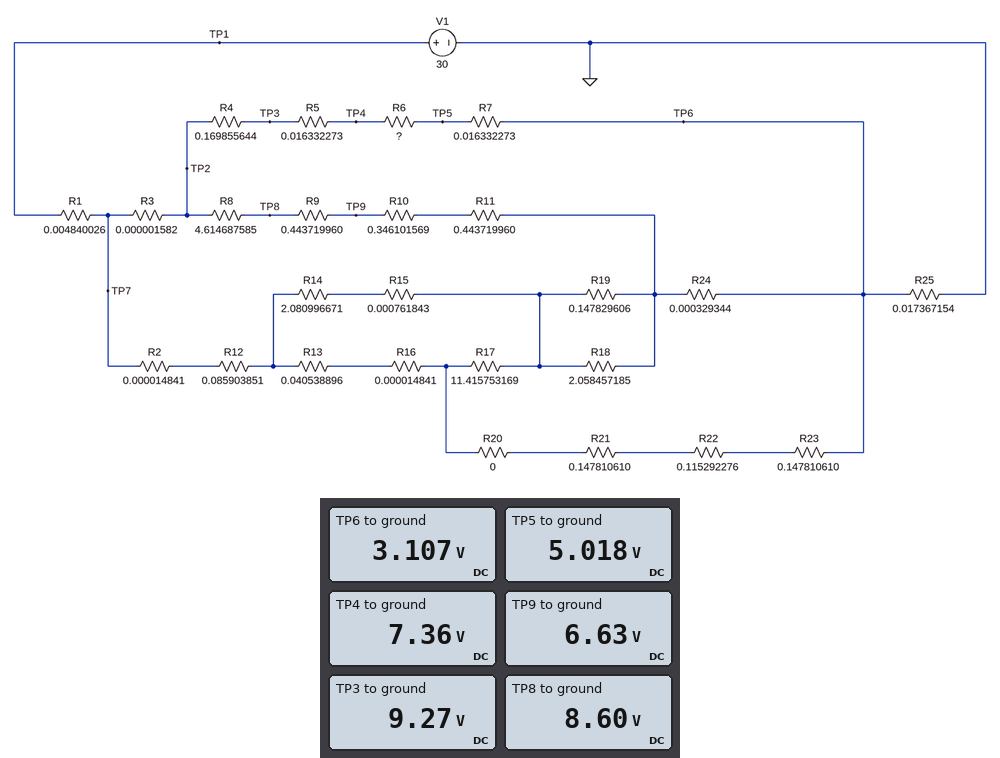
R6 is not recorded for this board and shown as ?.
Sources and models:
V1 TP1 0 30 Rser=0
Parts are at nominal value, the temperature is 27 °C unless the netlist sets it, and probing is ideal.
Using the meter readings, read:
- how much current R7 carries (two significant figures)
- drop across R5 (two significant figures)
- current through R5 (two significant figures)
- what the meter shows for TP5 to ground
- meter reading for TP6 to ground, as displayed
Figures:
120 A
1.9 V
120 A
5.018 V
3.107 V
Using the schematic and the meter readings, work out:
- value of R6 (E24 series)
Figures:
0.02 Ω
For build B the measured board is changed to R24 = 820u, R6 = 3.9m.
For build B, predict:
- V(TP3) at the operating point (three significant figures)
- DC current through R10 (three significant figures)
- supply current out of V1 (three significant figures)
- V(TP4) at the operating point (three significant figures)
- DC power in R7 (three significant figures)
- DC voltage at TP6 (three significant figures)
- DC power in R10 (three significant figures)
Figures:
7.82 V
4.42 A
187 A
5.78 V
256 W
3.24 V
6.76 W
